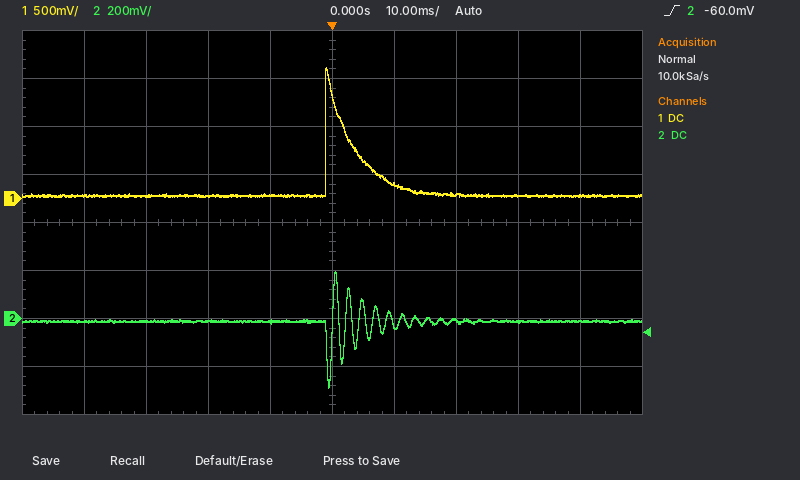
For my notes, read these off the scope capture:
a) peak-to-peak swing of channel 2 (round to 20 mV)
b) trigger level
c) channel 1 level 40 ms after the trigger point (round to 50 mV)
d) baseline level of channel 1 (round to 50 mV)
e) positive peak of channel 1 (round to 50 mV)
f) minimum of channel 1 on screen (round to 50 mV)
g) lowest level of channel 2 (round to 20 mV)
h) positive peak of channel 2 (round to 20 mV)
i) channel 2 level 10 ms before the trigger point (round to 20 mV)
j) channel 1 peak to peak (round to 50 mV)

480 mV
-60.0 mV
50 mV
50 mV
1.35 V
0 mV
-280 mV
200 mV
-20 mV
1.35 V
